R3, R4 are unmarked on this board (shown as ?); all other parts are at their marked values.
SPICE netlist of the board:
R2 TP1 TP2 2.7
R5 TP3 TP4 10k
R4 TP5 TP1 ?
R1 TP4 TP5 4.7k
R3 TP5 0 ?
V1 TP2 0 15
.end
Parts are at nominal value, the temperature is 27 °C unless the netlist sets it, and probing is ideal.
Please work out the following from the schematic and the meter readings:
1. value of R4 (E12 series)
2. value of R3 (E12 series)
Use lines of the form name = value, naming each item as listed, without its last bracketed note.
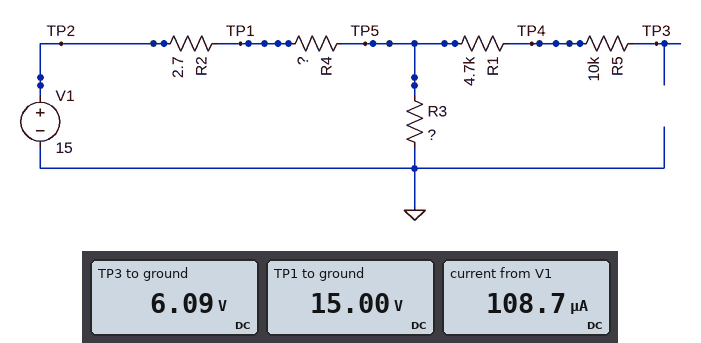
value of R4 = 82 kΩ
value of R3 = 56 kΩ
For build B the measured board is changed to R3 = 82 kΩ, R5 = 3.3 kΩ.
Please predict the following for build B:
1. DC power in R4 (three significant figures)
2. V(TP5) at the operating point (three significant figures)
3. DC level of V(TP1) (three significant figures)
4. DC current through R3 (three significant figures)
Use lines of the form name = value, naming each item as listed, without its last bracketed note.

DC power in R4 = 686 µW
V(TP5) at the operating point = 7.50 V
DC level of V(TP1) = 15.0 V
DC current through R3 = 91.5 µA
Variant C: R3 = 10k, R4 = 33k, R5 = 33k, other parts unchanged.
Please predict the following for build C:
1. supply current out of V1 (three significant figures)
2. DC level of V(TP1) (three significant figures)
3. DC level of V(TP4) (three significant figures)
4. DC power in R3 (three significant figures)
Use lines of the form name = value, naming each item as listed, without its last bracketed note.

supply current out of V1 = 349 µA
DC level of V(TP1) = 15.0 V
DC level of V(TP4) = 3.49 V
DC power in R3 = 1.22 mW
